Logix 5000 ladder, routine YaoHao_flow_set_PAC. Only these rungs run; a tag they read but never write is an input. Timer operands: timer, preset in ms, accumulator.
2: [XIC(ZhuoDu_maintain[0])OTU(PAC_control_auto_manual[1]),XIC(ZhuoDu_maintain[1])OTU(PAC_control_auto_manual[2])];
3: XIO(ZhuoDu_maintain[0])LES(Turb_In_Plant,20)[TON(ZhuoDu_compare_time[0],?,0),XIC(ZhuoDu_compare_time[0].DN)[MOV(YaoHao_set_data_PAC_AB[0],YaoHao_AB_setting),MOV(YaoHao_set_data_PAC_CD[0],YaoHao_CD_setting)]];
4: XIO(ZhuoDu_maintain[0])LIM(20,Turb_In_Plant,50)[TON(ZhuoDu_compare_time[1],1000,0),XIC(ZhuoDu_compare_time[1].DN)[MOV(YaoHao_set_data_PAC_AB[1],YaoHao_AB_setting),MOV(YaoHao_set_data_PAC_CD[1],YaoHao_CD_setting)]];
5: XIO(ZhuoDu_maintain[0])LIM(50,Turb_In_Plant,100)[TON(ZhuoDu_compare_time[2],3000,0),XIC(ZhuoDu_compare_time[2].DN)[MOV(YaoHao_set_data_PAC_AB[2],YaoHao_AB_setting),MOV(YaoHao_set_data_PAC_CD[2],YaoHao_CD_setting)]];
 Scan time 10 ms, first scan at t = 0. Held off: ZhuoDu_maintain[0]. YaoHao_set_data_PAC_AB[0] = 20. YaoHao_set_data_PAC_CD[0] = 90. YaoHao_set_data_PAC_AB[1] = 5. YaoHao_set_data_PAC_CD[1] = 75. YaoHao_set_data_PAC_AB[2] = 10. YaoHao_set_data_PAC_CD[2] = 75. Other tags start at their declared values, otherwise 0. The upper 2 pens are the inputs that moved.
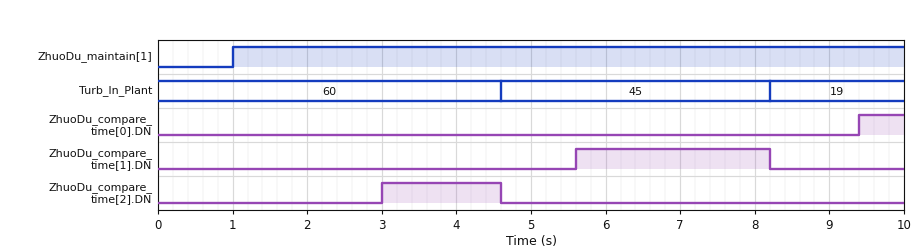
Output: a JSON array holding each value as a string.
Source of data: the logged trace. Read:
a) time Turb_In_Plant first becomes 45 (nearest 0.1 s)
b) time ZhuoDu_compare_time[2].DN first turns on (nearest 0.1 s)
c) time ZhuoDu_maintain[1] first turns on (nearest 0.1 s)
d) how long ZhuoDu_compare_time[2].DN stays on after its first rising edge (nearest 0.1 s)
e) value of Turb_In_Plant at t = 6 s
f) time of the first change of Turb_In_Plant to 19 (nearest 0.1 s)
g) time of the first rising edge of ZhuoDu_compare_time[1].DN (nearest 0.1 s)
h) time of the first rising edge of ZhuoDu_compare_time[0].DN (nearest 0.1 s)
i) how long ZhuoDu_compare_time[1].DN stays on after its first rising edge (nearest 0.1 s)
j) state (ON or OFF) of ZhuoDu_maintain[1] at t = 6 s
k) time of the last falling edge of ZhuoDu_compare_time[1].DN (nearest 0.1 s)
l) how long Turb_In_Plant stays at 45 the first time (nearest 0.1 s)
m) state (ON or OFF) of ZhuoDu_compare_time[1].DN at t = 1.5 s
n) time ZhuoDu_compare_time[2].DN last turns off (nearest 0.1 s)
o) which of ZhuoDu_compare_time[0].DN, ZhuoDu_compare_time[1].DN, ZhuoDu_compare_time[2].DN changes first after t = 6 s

["4.6 s", "3.0 s", "1.0 s", "1.6 s", "45", "8.2 s", "5.6 s", "9.4 s", "2.6 s", "ON", "8.2 s", "3.6 s", "OFF", "4.6 s", "ZhuoDu_compare_time[1].DN"]
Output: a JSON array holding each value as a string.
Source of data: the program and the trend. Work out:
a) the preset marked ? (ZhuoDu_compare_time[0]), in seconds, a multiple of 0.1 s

["1.2 s"]
